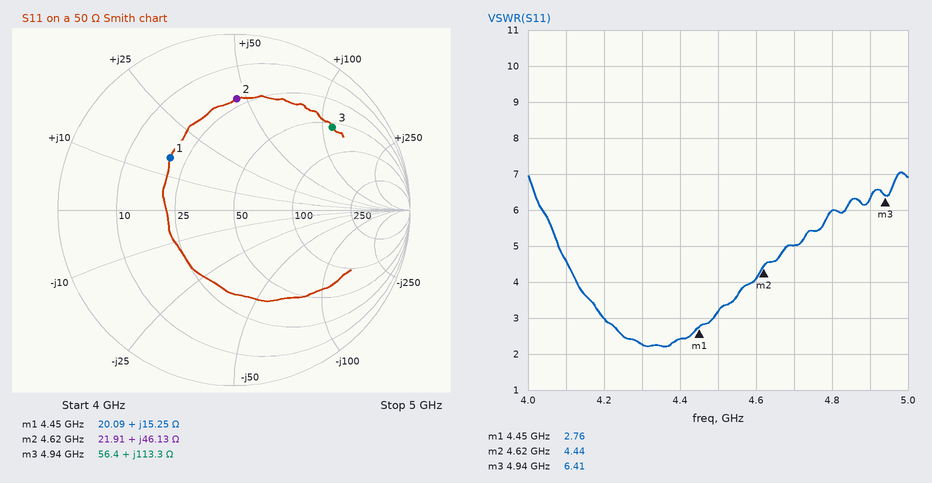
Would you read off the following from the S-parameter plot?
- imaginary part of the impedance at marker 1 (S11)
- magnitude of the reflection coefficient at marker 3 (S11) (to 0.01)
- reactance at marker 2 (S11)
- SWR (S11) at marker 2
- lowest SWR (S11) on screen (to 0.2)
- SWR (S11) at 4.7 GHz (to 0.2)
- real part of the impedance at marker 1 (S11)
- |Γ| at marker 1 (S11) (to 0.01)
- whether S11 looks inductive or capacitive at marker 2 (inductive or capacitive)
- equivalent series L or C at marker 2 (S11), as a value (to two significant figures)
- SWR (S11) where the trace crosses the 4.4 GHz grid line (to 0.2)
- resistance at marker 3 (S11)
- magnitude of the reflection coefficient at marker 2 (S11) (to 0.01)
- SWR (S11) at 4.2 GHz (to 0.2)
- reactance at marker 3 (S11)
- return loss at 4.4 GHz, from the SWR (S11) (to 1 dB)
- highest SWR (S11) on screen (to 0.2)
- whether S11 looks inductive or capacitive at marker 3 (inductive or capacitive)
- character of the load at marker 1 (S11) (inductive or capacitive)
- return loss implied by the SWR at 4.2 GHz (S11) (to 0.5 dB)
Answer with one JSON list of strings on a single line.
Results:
["+15.25 Ω", "0.73", "+46.13 Ω", "4.44", "2.2", "5.0", "20.09 Ω", "0.47", "inductive", "1.6 nH", "2.4", "56.4 Ω", "0.63", "3.0", "+113.3 Ω", "8 dB", "7.0", "inductive", "inductive", "6.0 dB"]
